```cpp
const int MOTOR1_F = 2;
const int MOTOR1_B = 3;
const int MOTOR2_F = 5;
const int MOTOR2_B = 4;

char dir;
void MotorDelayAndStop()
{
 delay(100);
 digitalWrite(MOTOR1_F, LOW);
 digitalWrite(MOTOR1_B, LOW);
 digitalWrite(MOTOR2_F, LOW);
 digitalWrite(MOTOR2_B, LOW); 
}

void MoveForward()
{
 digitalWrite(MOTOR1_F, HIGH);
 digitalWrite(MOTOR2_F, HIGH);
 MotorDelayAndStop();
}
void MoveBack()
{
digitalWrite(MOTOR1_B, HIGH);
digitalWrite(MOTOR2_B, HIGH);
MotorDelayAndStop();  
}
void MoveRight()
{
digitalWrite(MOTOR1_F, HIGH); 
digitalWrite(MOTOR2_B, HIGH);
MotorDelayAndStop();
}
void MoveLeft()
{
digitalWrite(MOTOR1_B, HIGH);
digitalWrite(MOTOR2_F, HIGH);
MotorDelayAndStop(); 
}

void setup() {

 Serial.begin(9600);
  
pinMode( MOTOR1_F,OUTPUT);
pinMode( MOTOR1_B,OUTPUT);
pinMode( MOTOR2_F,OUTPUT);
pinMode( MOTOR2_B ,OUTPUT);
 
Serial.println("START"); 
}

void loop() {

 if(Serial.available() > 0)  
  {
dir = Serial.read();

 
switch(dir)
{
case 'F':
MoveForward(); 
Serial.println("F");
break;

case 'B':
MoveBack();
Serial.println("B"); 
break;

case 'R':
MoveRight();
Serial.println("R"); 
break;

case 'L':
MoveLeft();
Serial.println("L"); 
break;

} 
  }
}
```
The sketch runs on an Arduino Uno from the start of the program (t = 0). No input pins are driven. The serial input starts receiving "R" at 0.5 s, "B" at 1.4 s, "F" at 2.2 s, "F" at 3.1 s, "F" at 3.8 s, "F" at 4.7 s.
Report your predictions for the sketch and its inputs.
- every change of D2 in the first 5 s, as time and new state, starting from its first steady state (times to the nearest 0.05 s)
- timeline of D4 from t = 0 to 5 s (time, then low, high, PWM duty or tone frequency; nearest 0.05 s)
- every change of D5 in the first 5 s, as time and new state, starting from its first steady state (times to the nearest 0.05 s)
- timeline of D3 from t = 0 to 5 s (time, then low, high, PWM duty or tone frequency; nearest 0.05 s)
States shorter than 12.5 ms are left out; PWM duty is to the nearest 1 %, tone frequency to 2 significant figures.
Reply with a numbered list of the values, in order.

1. 0 s low; 0.5 s high; 0.6 s low; 2.2 s high; 2.3 s low; 3.1 s high; 3.2 s low; 3.8 s high; 3.9 s low; 4.7 s high; 4.8 s low
2. 0 s low; 0.5 s high; 0.6 s low; 1.4 s high; 1.5 s low
3. 0 s low; 2.2 s high; 2.3 s low; 3.1 s high; 3.2 s low; 3.8 s high; 3.9 s low; 4.7 s high; 4.8 s low
4. 0 s low; 1.4 s high; 1.5 s low
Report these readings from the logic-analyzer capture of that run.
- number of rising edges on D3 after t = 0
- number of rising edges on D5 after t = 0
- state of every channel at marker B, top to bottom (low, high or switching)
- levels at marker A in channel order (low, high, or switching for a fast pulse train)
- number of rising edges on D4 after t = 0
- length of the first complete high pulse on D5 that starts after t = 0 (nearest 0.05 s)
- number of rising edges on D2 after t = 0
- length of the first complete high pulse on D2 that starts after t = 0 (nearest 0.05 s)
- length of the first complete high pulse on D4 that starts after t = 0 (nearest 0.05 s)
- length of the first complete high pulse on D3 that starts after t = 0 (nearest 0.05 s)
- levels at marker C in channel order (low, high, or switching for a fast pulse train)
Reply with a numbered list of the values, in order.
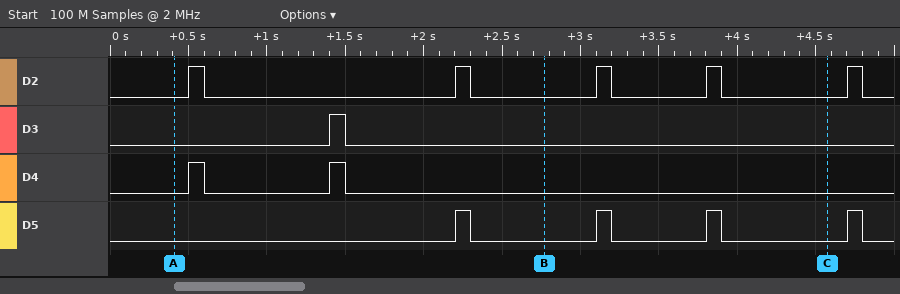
1. 1
2. 4
3. D2 low, D3 low, D4 low, D5 low
4. D2 low, D3 low, D4 low, D5 low
5. 2
6. 0.10 s
7. 5
8. 0.10 s
9. 0.10 s
10. 0.10 s
11. D2 low, D3 low, D4 low, D5 low
